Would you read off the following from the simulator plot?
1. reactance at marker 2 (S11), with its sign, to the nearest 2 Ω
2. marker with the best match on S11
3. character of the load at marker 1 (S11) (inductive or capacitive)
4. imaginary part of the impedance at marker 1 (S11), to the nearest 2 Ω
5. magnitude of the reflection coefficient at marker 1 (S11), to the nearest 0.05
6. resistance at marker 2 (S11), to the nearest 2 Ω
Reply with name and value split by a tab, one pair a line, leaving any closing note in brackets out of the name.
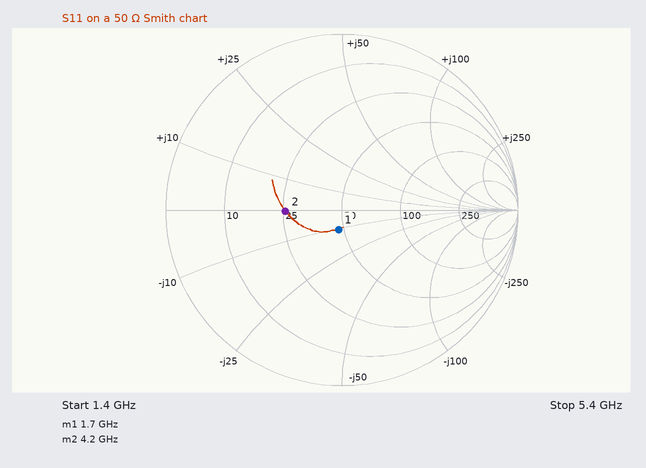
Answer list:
reactance at marker 2 (S11), with its sign, to the nearest 2 Ω	0 Ω
marker with the best match on S11	marker 1
character of the load at marker 1 (S11)	capacitive
imaginary part of the impedance at marker 1 (S11), to the nearest 2 Ω	-10 Ω
magnitude of the reflection coefficient at marker 1 (S11), to the nearest 0.05	0.10
resistance at marker 2 (S11), to the nearest 2 Ω	26 Ω
